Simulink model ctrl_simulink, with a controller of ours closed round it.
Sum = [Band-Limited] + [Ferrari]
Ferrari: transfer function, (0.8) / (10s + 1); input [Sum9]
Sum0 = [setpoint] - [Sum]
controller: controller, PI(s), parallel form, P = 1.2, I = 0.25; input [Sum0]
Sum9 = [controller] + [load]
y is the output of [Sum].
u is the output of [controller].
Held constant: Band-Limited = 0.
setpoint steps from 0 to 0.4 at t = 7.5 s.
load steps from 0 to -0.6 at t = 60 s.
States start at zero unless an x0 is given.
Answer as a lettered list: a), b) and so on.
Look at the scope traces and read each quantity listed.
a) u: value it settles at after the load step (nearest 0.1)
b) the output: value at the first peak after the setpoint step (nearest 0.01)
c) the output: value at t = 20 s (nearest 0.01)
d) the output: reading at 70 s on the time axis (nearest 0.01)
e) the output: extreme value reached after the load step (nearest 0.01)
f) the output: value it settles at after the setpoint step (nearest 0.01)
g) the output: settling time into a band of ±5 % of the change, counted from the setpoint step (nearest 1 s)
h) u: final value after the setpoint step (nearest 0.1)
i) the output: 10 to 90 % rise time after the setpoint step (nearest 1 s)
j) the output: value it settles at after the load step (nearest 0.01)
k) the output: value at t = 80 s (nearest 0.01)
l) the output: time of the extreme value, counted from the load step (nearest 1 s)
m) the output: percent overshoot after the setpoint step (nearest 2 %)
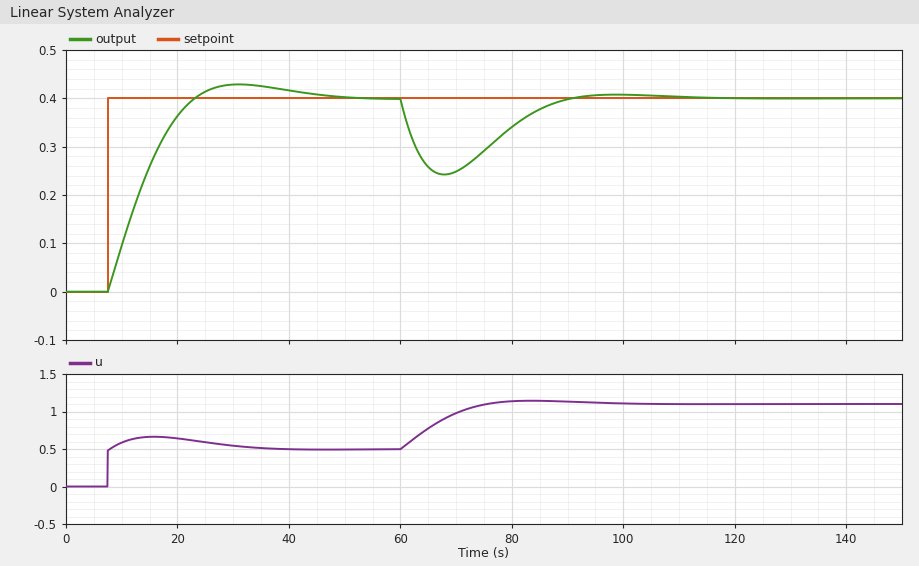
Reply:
a) 1.1
b) 0.43
c) 0.36
d) 0.25
e) 0.24
f) 0.40
g) 31 s
h) 0.5
i) 11 s
j) 0.40
k) 0.34
l) 8 s
m) 8 %
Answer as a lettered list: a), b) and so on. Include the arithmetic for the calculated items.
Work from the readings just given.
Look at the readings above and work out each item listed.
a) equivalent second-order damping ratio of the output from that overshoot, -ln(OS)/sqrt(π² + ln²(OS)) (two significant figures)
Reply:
a) ln(0.08) = -2.526; 2.526 / sqrt(9.870 + 6.379) = 0.63
